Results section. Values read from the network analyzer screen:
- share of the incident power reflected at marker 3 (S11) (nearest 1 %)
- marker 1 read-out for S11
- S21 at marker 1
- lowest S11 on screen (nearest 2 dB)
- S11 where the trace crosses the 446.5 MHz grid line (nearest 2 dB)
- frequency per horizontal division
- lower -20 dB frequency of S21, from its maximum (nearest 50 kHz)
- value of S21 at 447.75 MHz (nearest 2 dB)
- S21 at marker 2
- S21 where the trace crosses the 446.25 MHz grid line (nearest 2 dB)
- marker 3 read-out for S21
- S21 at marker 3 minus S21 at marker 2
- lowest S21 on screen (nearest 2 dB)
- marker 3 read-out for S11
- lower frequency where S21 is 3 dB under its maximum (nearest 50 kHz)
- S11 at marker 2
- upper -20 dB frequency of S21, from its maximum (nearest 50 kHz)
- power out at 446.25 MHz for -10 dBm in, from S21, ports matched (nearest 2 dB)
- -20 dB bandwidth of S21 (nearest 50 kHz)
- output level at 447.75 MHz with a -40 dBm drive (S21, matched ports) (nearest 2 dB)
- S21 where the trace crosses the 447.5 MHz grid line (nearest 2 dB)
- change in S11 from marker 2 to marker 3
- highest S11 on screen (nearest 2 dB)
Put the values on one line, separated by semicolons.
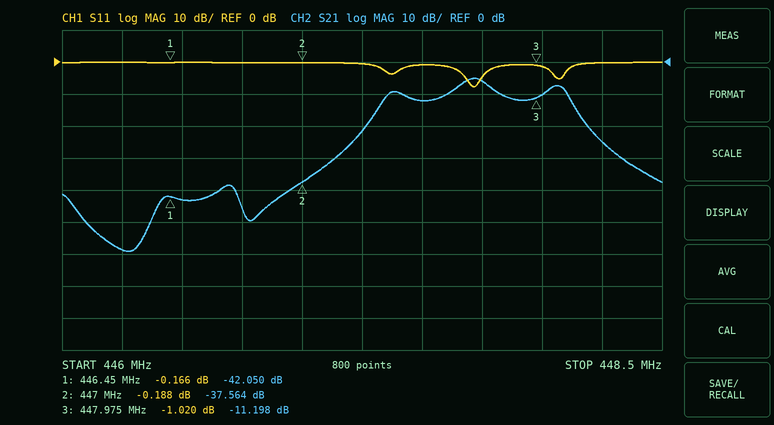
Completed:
79 %; -0.166 dB; -42.050 dB; -8 dB; 0 dB; 250 kHz; 447.20 MHz; -6 dB; -37.564 dB; -58 dB; -11.198 dB; 26.366 dB; -60 dB; -1.020 dB; 447.65 MHz; -0.188 dB; 448.25 MHz; -68 dBm; 1.05 MHz; -46 dBm; -12 dB; -0.832 dB; 0 dB
